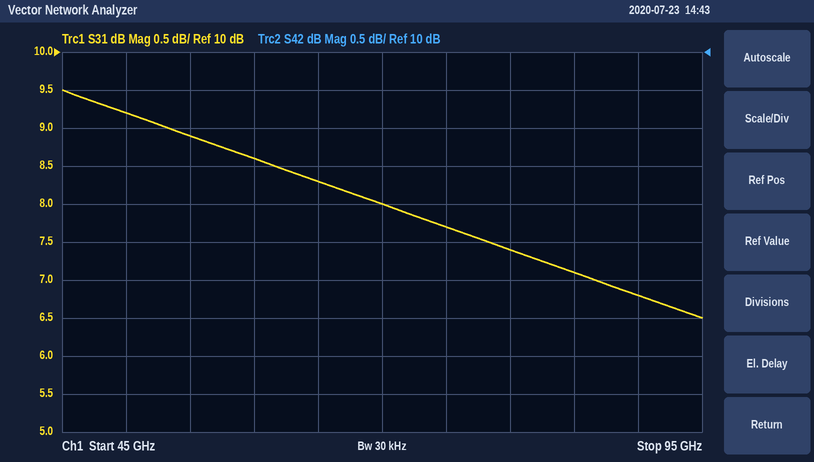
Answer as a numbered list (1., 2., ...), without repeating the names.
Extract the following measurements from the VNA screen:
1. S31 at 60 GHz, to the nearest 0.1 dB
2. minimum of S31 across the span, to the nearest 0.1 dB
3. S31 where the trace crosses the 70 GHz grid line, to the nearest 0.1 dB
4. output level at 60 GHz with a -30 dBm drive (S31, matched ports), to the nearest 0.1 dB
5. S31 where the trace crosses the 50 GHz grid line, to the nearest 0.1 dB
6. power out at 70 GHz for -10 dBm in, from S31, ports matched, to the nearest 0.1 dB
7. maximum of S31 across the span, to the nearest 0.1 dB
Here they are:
1. 8.6 dB
2. 6.5 dB
3. 8.0 dB
4. -21.4 dBm
5. 9.2 dB
6. -2.0 dBm
7. 9.5 dB
